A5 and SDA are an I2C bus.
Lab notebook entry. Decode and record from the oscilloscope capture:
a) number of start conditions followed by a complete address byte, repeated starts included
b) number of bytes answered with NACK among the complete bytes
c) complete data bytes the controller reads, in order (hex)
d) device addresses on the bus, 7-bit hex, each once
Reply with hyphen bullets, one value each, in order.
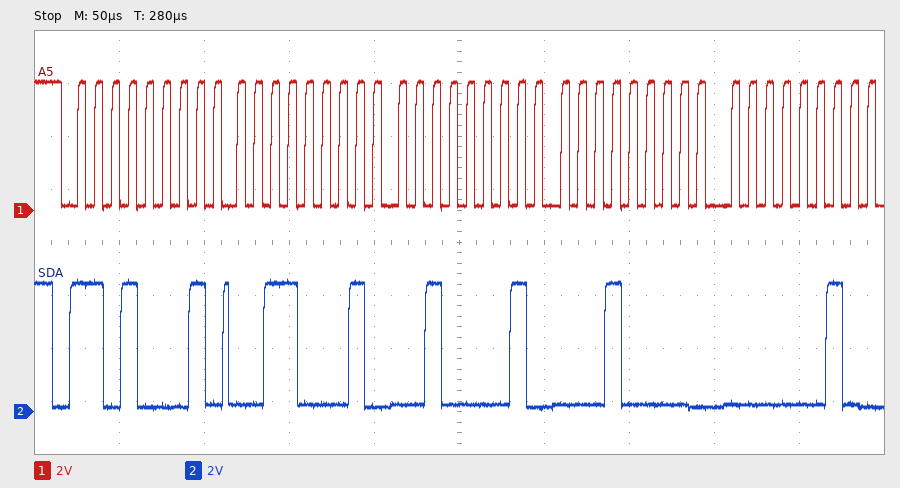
- 1
- 0
- 31 21 10 02
- 0x68
